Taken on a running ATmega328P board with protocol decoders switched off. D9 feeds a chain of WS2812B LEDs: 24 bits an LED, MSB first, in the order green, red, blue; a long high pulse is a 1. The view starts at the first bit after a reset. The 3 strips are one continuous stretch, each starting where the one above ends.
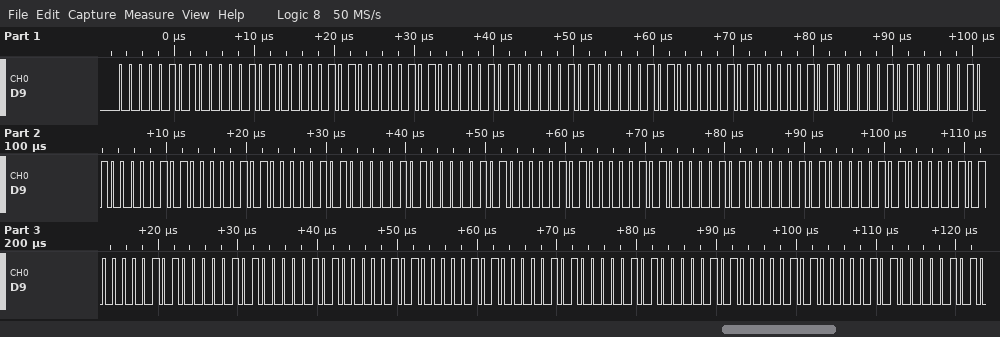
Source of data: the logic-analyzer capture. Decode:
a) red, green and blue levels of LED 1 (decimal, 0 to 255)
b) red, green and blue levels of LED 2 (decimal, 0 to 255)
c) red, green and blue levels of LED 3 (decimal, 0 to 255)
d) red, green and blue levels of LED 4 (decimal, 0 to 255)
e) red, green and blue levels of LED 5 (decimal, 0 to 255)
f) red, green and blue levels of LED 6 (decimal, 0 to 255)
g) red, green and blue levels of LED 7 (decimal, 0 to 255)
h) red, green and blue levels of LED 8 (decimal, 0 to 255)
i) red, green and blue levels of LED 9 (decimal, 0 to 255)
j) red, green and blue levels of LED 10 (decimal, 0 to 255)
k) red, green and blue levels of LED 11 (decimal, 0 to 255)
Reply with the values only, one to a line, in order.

5, 5, 5
5, 5, 5
5, 5, 5
5, 5, 5
5, 5, 5
5, 5, 5
5, 5, 5
5, 5, 5
5, 5, 5
5, 5, 5
5, 5, 5
